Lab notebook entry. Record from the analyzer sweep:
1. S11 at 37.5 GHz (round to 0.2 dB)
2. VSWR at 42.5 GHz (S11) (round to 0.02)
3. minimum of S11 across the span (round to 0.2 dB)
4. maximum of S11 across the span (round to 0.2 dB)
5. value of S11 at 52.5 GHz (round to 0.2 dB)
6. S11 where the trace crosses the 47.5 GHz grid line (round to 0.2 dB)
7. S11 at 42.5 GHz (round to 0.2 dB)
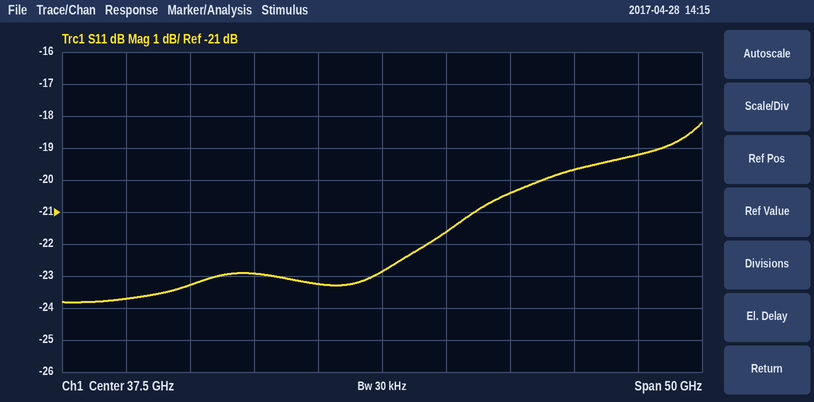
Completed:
-22.8 dB
1.18
-23.8 dB
-18.2 dB
-19.6 dB
-20.4 dB
-21.6 dB
